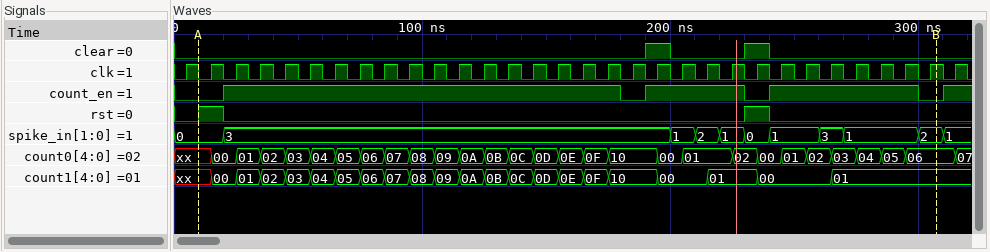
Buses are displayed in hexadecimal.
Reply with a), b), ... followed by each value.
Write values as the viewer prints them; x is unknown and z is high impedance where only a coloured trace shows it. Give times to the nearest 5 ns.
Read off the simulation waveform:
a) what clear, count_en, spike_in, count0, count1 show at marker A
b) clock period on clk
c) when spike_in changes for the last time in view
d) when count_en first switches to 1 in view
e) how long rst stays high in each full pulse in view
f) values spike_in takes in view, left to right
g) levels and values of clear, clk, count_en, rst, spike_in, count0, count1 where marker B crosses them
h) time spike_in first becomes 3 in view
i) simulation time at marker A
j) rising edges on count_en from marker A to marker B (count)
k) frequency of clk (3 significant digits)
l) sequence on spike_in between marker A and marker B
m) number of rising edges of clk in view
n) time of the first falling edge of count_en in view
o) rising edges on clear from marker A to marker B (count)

a) clear=0, count_en=0, spike_in=0, count0=xx, count1=xx
b) 10 ns
c) 310 ns
d) 20 ns
e) 10 ns, 10 ns
f) 0, 3, 1, 2, 1, 0, 1, 3, 1, 2, 1
g) clear=0, clk=1, count_en=0, rst=0, spike_in=2, count0=06, count1=01
h) 20 ns
i) 10 ns
j) 3
k) 100 MHz
l) 0, 3, 1, 2, 1, 0, 1, 3, 1, 2
m) 32
n) 180 ns
o) 2
